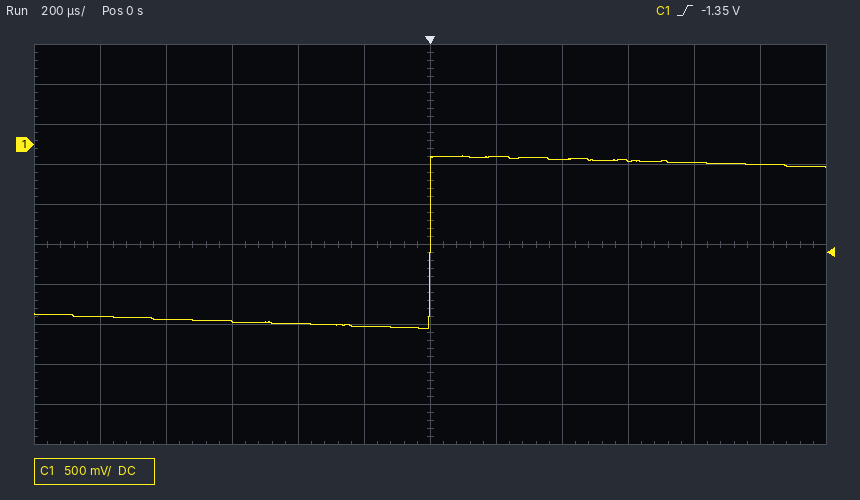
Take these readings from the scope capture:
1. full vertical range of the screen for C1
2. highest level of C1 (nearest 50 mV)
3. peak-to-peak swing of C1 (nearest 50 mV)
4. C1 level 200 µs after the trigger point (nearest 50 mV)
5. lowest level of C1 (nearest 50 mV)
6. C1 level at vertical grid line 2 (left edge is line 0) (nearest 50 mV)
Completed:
5 V
-150 mV
2.15 V
-150 mV
-2.30 V
-2.20 V
